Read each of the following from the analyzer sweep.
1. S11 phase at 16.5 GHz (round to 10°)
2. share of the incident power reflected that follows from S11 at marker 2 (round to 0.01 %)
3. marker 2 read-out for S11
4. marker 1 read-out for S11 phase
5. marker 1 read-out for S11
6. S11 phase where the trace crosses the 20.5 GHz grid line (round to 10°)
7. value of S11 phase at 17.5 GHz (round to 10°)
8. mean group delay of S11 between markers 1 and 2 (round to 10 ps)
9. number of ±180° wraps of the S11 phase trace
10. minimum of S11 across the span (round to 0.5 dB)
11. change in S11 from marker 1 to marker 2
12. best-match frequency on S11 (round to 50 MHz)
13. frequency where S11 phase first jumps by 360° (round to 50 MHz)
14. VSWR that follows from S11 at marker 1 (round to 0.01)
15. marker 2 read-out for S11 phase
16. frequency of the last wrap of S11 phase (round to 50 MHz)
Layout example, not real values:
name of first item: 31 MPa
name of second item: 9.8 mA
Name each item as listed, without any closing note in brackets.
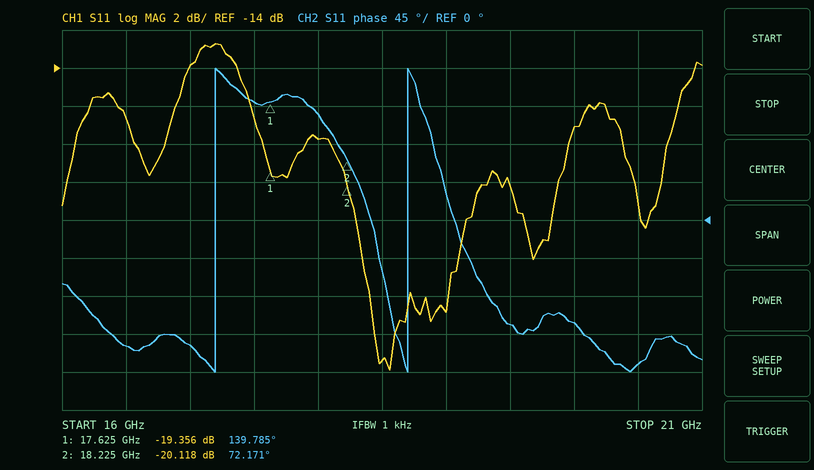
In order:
S11 phase at 16.5 GHz: -150°
share of the incident power reflected that follows from S11 at marker 2: 0.97 %
marker 2 read-out for S11: -20.118 dB
marker 1 read-out for S11 phase: 139.785°
marker 1 read-out for S11: -19.356 dB
S11 phase where the trace crosses the 20.5 GHz grid line: -170°
value of S11 phase at 17.5 GHz: 140°
mean group delay of S11 between markers 1 and 2: 310 ps
number of ±180° wraps of the S11 phase trace: 2
minimum of S11 across the span: -30.0 dB
change in S11 from marker 1 to marker 2: -0.762 dB
best-match frequency on S11: 18.55 GHz
frequency where S11 phase first jumps by 360°: 17.20 GHz
VSWR that follows from S11 at marker 1: 1.24
marker 2 read-out for S11 phase: 72.171°
frequency of the last wrap of S11 phase: 18.70 GHz
